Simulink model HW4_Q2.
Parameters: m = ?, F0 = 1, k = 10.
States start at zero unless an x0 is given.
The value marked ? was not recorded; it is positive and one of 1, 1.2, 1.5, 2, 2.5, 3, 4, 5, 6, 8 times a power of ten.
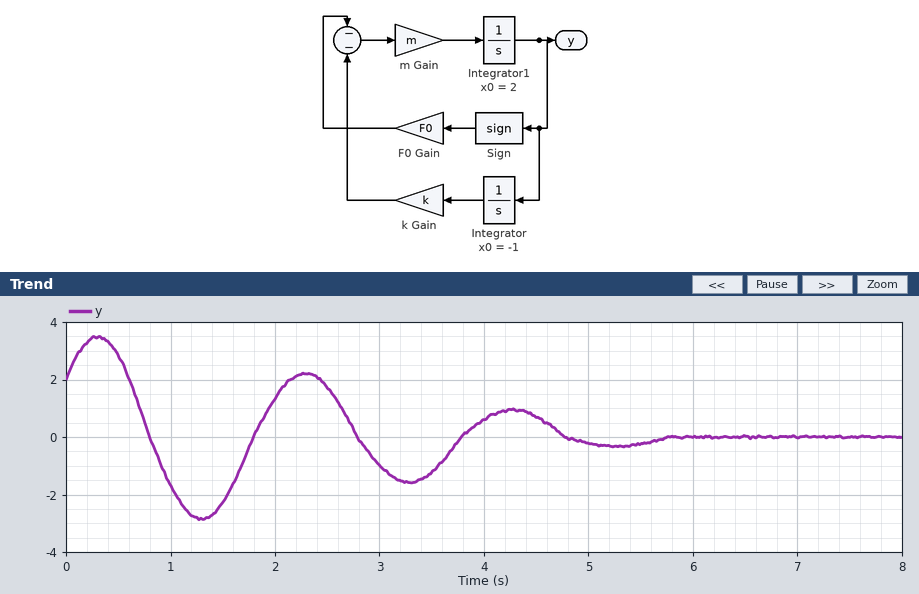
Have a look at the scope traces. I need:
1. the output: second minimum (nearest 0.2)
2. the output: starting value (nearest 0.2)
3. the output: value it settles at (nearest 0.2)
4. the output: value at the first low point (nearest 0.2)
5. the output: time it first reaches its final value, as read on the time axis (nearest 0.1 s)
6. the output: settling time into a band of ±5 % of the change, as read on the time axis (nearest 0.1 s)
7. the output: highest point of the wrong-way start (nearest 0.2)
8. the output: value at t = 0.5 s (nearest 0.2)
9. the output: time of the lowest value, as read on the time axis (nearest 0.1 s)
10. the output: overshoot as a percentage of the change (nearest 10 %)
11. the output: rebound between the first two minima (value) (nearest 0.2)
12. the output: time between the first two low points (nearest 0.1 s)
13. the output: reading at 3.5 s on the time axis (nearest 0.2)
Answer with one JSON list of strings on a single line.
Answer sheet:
["-1.6", "2.0", "0.0", "-2.8", "0.8 s", "5.7 s", "3.4", "2.8", "1.3 s", "140 %", "2.2", "2.0 s", "-1.2"]
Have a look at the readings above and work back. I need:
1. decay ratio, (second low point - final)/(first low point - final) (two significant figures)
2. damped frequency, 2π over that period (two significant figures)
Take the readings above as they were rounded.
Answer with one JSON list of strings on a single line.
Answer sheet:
["0.57", "3.1 rad/s"]
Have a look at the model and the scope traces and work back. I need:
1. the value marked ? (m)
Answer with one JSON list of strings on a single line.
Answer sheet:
["1"]
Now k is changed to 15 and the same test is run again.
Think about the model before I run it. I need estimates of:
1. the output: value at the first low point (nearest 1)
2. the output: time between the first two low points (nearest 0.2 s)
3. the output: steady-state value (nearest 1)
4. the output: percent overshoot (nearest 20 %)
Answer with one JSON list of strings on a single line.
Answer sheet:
["-4", "1.6 s", "0", "180 %"]
